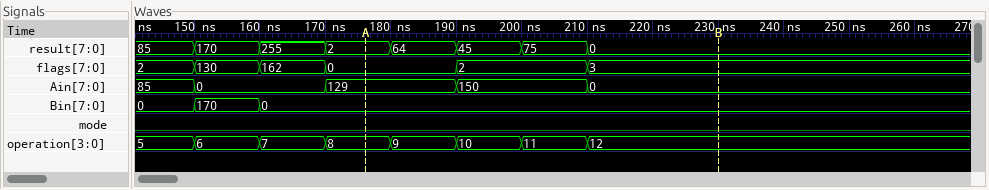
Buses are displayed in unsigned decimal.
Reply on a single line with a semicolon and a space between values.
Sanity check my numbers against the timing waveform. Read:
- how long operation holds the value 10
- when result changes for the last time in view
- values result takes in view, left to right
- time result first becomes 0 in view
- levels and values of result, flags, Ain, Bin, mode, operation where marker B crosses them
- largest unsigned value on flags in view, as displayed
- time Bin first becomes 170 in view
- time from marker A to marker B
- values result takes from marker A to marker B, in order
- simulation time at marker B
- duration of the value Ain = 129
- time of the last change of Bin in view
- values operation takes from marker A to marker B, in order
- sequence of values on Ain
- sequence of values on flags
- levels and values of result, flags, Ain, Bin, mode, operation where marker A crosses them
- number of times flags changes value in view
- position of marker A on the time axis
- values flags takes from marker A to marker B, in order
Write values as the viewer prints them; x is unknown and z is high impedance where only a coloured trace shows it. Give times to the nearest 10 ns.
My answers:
10 ns; 210 ns; 85, 170, 255, 2, 64, 45, 75, 0; 210 ns; result=0, flags=3, Ain=0, Bin=0, mode=0, operation=12; 162; 150 ns; 50 ns; 2, 64, 45, 75, 0; 230 ns; 20 ns; 160 ns; 8, 9, 10, 11, 12; 85, 0, 129, 150, 0; 2, 130, 162, 0, 2, 3; result=2, flags=0, Ain=129, Bin=0, mode=0, operation=8; 5; 180 ns; 0, 2, 3
